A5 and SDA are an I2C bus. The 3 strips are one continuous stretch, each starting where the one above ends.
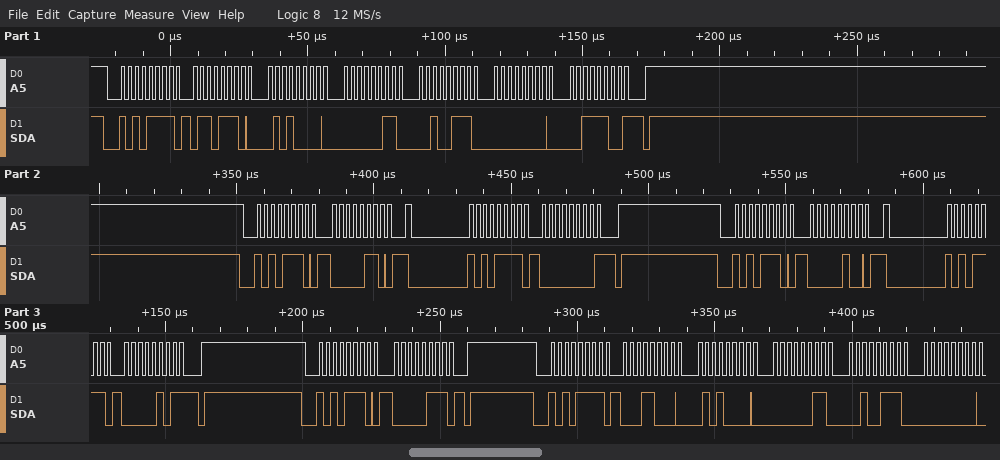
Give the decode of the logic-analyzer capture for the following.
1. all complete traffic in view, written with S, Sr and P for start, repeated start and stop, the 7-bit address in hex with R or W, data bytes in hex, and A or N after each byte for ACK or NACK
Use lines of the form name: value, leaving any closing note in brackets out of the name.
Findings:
all complete traffic in view, written with S, Sr and P for start, repeated start and stop, the 7-bit address in hex with R or W, data bytes in hex, and A or N after each byte for ACK or NACK: S 57R A 6E A 50 A 03 A 27 A 00 A 3C N P S 57W A 06 A Sr 57R A 00 N P S 57W A 04 A Sr 57R A 05 N P S 57W A 07 A P S 57R A 18 A 50 A 03 A 27 A 00 A
